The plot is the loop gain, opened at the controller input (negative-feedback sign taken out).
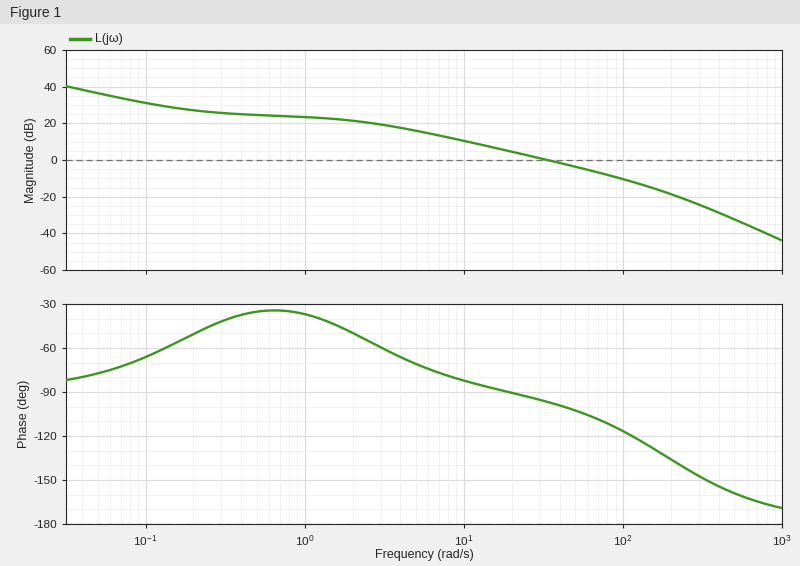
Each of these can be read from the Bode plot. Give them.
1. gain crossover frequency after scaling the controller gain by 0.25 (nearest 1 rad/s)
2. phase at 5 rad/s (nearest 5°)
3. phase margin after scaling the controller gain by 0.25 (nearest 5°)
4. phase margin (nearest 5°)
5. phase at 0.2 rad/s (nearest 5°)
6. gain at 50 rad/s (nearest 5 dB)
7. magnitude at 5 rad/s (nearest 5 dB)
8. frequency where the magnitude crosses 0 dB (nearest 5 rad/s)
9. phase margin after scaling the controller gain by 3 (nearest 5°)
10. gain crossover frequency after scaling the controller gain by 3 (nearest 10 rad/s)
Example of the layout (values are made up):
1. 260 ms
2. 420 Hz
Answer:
1. 8 rad/s
2. -70°
3. 100°
4. 85°
5. -50°
6. -5 dB
7. 15 dB
8. 35 rad/s
9. 65°
10. 90 rad/s
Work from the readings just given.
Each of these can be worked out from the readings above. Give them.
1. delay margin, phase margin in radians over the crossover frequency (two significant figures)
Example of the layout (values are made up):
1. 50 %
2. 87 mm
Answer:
1. 0.042 s
